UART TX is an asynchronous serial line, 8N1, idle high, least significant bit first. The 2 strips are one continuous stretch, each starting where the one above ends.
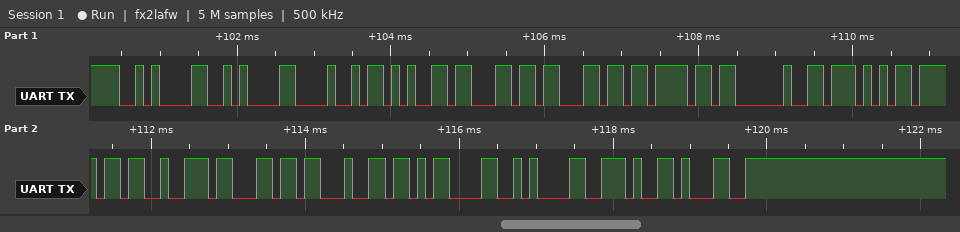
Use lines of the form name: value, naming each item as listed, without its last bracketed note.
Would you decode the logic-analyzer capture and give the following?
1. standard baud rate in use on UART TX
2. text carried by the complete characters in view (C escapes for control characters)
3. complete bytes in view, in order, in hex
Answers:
standard baud rate in use on UART TX: 9600 baud
text carried by the complete characters in view: "\n\nHello World\r\n.1"
complete bytes in view, in order, in hex: 0A 0A 48 65 6C 6C 6F 20 57 6F 72 6C 64 0D 0A 2E 31
